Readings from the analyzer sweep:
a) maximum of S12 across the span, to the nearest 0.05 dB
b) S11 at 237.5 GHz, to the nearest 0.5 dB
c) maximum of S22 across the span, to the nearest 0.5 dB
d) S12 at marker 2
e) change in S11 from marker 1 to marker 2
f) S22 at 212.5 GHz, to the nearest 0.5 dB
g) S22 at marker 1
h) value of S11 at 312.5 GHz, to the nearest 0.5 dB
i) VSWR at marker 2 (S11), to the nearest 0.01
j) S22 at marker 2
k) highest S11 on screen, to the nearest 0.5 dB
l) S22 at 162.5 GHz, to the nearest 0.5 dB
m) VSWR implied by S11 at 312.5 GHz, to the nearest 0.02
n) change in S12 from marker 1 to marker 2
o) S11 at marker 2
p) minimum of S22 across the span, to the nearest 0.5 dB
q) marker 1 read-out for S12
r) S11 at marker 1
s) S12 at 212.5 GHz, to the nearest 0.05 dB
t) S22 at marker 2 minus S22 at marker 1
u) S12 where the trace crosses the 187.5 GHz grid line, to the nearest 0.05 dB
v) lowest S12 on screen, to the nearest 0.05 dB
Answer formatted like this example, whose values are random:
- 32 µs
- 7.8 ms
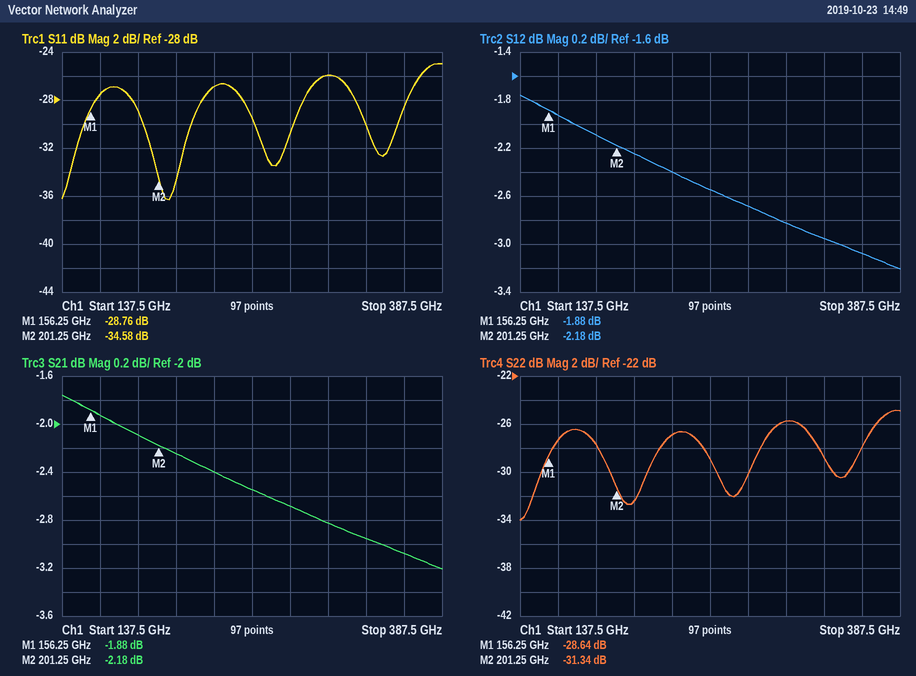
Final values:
- -1.75 dB
- -27.0 dB
- -25.0 dB
- -2.18 dB
- -5.82 dB
- -32.5 dB
- -28.64 dB
- -26.0 dB
- 1.04
- -31.34 dB
- -25.0 dB
- -27.5 dB
- 1.10
- -0.30 dB
- -34.58 dB
- -34.0 dB
- -1.88 dB
- -28.76 dB
- -2.25 dB
- -2.70 dB
- -2.10 dB
- -3.20 dB
